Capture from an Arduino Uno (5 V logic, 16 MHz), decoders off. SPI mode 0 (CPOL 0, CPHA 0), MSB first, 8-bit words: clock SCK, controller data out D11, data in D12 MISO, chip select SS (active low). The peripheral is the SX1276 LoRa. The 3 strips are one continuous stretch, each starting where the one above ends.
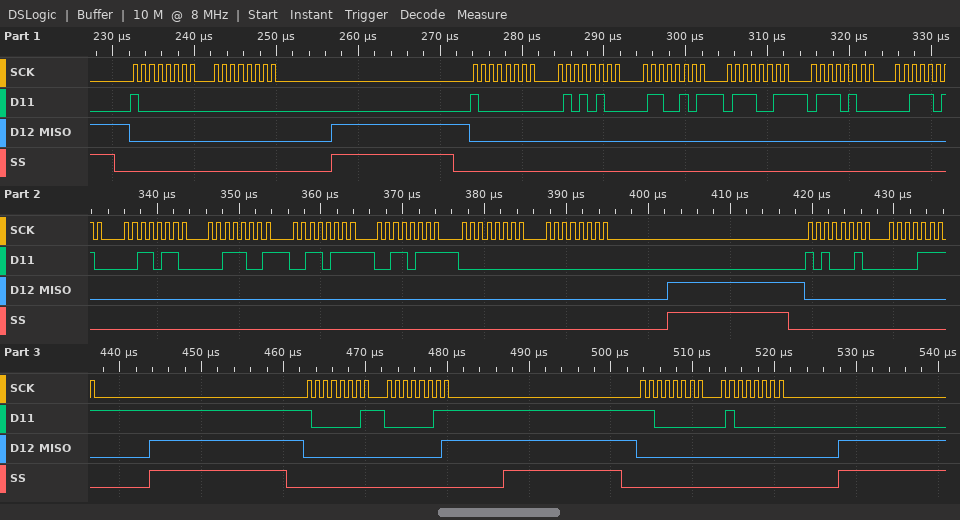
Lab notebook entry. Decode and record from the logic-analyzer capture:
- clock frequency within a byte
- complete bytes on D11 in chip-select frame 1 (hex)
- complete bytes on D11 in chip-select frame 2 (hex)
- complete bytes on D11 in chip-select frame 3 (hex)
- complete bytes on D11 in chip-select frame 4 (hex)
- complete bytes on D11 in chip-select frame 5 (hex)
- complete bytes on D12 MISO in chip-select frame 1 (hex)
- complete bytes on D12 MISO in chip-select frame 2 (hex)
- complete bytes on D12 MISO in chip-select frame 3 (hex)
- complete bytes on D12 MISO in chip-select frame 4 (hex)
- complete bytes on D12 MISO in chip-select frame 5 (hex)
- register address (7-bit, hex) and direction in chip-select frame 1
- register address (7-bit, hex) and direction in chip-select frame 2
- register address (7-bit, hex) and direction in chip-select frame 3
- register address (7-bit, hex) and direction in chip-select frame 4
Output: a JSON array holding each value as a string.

["1 MHz", "80 00", "80 54 65 73 74 3A 36 39 37 37 00 00", "A2 0F", "81 03", "C0 40", "00 00", "00 00 00 00 00 00 00 00 00 00 00 00", "00 00", "00 01", "00 00", "0x00 write", "0x00 write", "0x22 write", "0x01 write"]
